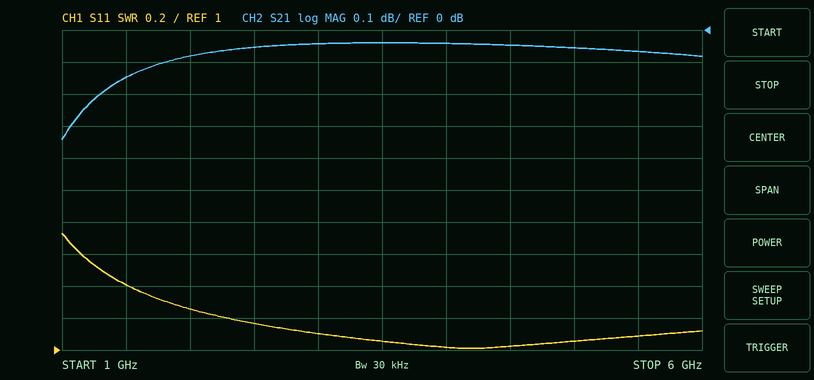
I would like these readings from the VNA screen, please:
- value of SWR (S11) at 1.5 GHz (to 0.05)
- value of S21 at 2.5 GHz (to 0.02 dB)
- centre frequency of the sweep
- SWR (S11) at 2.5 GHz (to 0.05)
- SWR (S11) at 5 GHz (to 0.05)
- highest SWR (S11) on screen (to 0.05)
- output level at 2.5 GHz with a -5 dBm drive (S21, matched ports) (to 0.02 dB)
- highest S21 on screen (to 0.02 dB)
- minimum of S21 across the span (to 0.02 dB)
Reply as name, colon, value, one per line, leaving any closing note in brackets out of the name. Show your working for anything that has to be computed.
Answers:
value of SWR (S11) at 1.5 GHz: 1.40
value of S21 at 2.5 GHz: -0.06 dB
centre frequency of the sweep: 3.5 GHz
SWR (S11) at 2.5 GHz: 1.15
SWR (S11) at 5 GHz: 1.05
highest SWR (S11) on screen: 1.75
output level at 2.5 GHz with a -5 dBm drive (S21, matched ports): -5 dBm + (-0.06 dB) = -5.06 dBm
highest S21 on screen: -0.04 dB
minimum of S21 across the span: -0.34 dB
